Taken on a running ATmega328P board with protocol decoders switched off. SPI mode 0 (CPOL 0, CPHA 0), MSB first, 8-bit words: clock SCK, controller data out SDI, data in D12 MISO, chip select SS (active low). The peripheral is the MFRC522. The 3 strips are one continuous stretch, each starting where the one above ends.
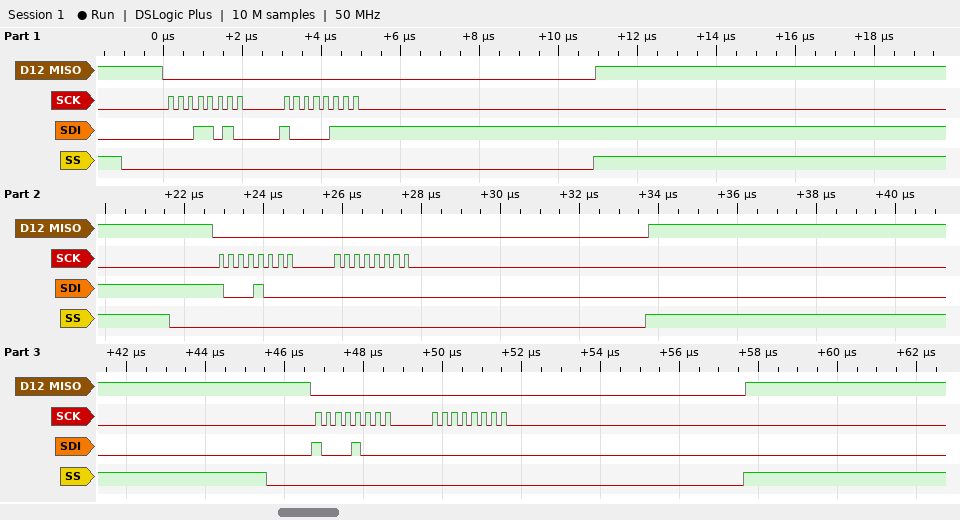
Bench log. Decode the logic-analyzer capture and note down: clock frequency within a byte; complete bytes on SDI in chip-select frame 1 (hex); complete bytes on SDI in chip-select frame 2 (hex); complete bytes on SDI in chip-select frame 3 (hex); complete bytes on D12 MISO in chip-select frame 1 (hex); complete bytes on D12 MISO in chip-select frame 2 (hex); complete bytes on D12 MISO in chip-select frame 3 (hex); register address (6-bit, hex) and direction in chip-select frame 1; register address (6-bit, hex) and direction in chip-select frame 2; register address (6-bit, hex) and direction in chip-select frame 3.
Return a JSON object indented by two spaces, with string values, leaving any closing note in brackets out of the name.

{
  "clock frequency within a byte": "4 MHz",
  "complete bytes on SDI in chip-select frame 1": "1A 87",
  "complete bytes on SDI in chip-select frame 2": "88 00",
  "complete bytes on SDI in chip-select frame 3": "88 00",
  "complete bytes on D12 MISO in chip-select frame 1": "00 00",
  "complete bytes on D12 MISO in chip-select frame 2": "00 00",
  "complete bytes on D12 MISO in chip-select frame 3": "00 00",
  "register address (6-bit, hex) and direction in chip-select frame 1": "0x0D write",
  "register address (6-bit, hex) and direction in chip-select frame 2": "0x04 read",
  "register address (6-bit, hex) and direction in chip-select frame 3": "0x04 read"
}
